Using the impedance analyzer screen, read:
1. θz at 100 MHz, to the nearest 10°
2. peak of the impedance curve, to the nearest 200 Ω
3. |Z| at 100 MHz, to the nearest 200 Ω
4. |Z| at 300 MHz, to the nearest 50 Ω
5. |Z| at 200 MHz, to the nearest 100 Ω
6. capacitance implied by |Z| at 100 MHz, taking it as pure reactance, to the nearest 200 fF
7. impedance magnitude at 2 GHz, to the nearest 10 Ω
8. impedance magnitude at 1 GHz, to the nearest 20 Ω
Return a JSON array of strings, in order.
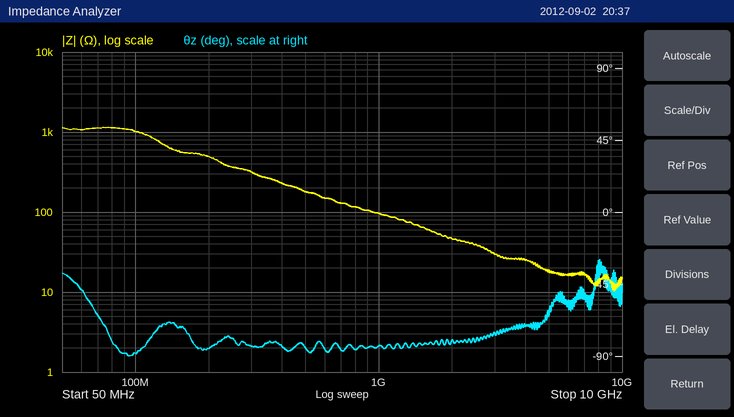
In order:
["-90°", "1.2 kΩ", "1.0 kΩ", "300 Ω", "500 Ω", "1.6 pF", "50 Ω", "100 Ω"]
